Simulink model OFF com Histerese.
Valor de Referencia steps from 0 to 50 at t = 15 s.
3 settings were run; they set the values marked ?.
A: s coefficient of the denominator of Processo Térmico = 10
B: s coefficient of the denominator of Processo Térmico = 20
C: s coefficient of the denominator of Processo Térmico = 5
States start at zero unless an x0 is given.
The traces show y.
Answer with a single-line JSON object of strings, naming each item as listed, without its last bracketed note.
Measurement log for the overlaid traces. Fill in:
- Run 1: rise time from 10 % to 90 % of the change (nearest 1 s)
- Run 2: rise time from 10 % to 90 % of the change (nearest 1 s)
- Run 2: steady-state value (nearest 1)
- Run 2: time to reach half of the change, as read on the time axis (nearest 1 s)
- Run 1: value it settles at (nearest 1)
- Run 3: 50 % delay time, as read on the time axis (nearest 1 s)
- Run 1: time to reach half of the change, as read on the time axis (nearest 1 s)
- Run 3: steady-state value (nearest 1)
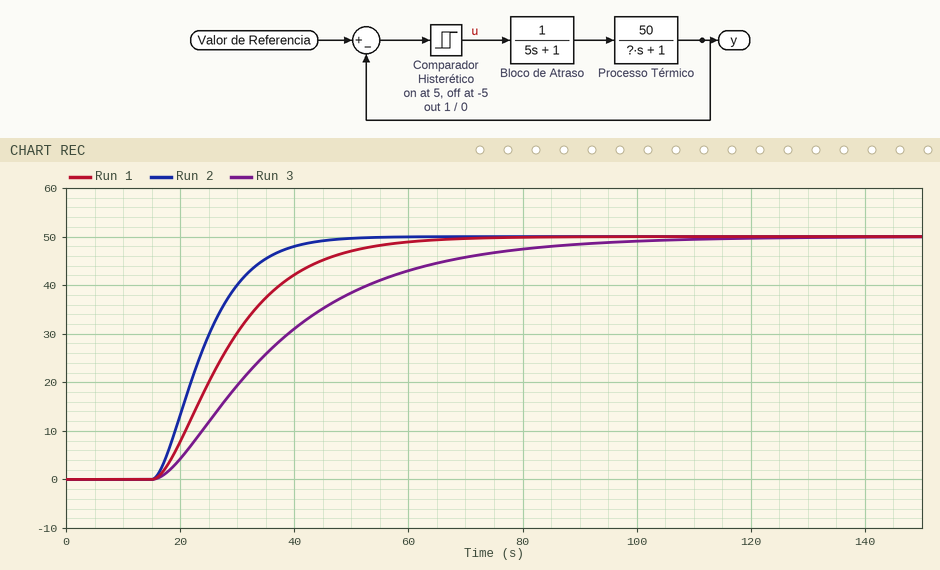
{"Run 1: rise time from 10 % to 90 % of the change": "26 s", "Run 2: rise time from 10 % to 90 % of the change": "17 s", "Run 2: steady-state value": "50", "Run 2: time to reach half of the change, as read on the time axis": "23 s", "Run 1: value it settles at": "50", "Run 3: 50 % delay time, as read on the time axis": "34 s", "Run 1: time to reach half of the change, as read on the time axis": "27 s", "Run 3: steady-state value": "50"}
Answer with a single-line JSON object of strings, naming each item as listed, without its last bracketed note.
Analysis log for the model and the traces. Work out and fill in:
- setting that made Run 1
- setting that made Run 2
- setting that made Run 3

{"setting that made Run 1": "A", "setting that made Run 2": "C", "setting that made Run 3": "B"}
